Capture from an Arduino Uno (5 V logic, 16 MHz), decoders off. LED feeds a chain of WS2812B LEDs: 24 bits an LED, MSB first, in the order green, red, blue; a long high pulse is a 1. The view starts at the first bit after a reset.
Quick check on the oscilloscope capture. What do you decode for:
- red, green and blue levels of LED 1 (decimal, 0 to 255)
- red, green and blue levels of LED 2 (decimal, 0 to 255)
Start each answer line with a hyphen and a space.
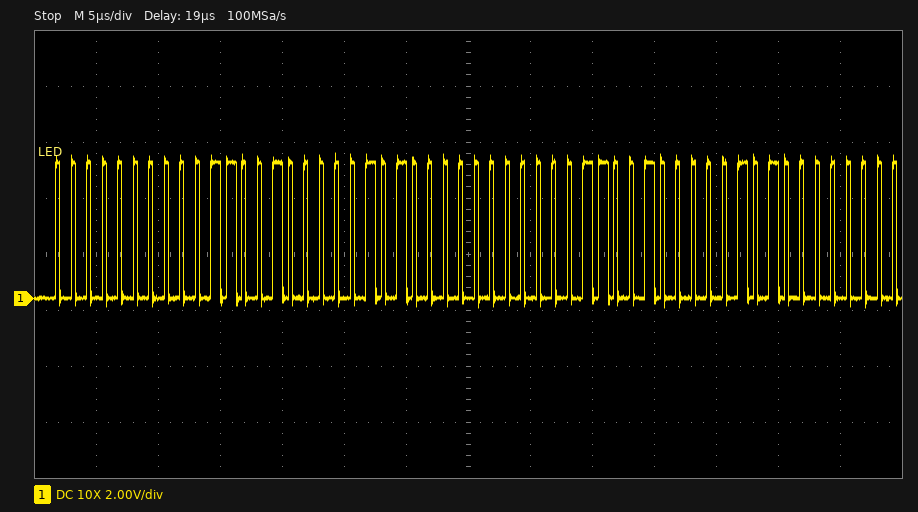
- 50, 0, 10
- 50, 0, 10
